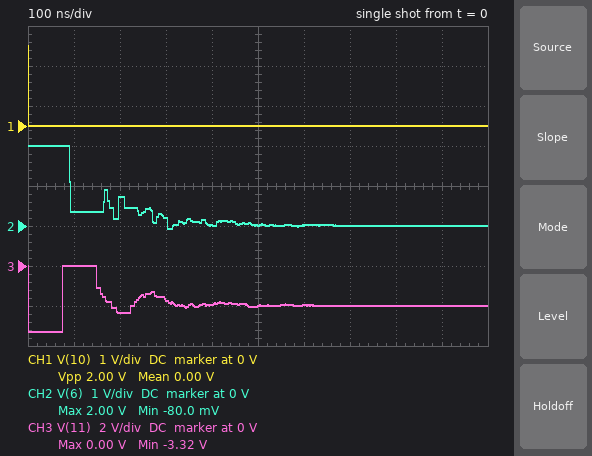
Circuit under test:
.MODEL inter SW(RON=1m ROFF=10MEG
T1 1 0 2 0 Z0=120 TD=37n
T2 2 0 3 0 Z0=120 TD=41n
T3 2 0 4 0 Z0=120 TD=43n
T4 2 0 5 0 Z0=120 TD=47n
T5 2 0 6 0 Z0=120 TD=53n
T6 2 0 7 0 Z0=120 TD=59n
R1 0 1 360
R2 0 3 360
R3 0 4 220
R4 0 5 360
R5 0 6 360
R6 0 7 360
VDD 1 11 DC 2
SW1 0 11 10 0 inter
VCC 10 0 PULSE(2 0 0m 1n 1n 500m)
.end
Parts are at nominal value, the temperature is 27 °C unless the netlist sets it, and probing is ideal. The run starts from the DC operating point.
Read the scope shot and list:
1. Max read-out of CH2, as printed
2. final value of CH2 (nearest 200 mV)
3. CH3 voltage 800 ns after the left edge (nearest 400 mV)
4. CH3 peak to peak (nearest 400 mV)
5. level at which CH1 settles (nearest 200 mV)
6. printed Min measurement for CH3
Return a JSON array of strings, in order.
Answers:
["2.00 V", "0 V", "-2.0 V", "3.2 V", "0 V", "-3.32 V"]
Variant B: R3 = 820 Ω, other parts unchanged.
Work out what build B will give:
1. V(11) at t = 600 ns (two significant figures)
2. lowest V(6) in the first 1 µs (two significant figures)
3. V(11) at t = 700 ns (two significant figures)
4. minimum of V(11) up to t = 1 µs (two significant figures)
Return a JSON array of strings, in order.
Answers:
["-1.9 V", "-2.9 mV", "-2.0 V", "-2.7 V"]
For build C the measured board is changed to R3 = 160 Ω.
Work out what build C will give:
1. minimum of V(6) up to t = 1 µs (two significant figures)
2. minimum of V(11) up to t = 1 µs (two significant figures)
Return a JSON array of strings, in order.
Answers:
["-150 mV", "-3.6 V"]
